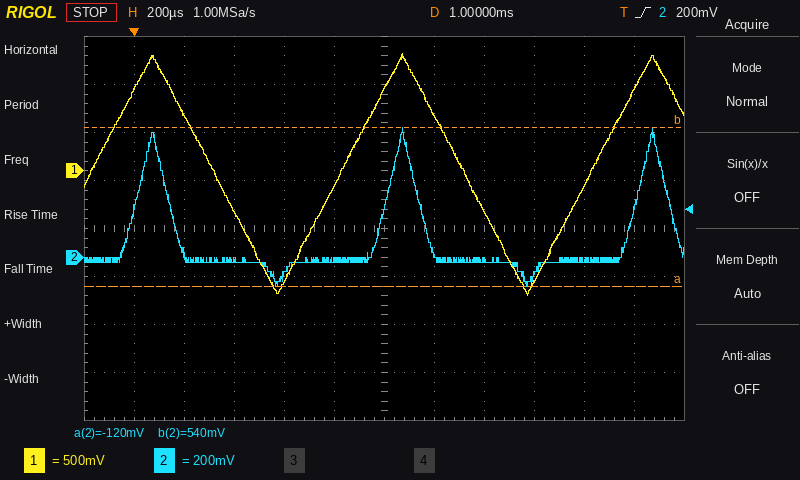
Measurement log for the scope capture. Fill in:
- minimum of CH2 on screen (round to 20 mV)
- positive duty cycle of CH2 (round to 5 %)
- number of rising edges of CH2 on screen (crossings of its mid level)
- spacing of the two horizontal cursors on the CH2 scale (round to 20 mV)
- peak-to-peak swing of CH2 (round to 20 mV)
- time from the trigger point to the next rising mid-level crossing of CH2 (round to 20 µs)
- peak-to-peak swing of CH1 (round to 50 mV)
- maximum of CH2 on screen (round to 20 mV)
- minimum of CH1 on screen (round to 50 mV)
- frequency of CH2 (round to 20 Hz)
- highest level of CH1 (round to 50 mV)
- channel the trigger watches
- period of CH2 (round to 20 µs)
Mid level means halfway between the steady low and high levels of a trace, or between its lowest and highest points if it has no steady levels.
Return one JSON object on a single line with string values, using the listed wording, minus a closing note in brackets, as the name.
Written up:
{"minimum of CH2 on screen": "-120 mV", "positive duty cycle of CH2": "15 %", "number of rising edges of CH2 on screen": "3", "spacing of the two horizontal cursors on the CH2 scale": "660 mV", "peak-to-peak swing of CH2": "660 mV", "time from the trigger point to the next rising mid-level crossing of CH2": "1.00 ms", "peak-to-peak swing of CH1": "2.50 V", "maximum of CH2 on screen": "540 mV", "minimum of CH1 on screen": "-1.30 V", "frequency of CH2": "1.00 kHz", "highest level of CH1": "1.20 V", "channel the trigger watches": "CH2", "period of CH2": "1.00 ms"}
